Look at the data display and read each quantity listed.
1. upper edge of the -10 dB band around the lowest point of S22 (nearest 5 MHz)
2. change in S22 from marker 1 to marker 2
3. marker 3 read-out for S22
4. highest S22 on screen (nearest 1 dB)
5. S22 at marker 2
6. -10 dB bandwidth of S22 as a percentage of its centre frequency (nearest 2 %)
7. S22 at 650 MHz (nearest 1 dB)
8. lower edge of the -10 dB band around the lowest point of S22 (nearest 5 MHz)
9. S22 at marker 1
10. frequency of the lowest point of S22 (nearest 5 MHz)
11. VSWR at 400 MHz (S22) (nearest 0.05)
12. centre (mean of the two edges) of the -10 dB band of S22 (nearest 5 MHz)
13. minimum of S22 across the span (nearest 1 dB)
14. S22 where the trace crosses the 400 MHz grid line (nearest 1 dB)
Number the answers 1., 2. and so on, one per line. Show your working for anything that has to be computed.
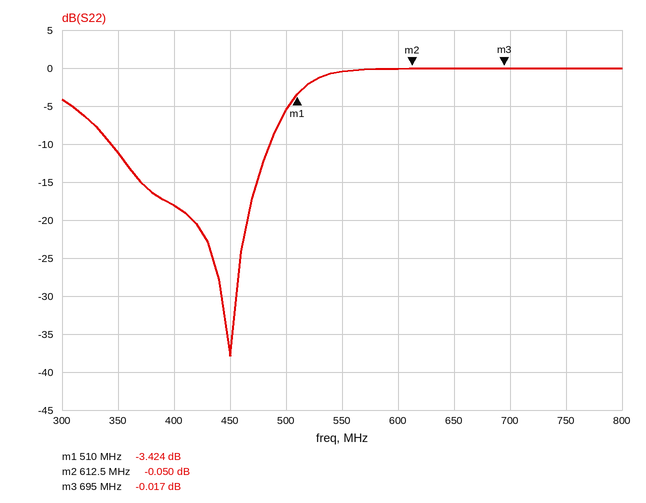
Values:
1. 485 MHz
2. -0.05 − (-3.424) = 3.374 dB
3. -0.017 dB
4. 0 dB
5. -0.050 dB
6. 140 MHz / 415 MHz ≈ 34 %
7. 0 dB
8. 345 MHz
9. -3.424 dB
10. 450 MHz
11. |Γ| = 10^(-18/20) = 0.1259; VSWR = (1 + 0.1259)/(1 − 0.1259) ≈ 1.29, so 1.30 to the nearest 0.05
12. 415 MHz
13. -38 dB
14. -18 dB
